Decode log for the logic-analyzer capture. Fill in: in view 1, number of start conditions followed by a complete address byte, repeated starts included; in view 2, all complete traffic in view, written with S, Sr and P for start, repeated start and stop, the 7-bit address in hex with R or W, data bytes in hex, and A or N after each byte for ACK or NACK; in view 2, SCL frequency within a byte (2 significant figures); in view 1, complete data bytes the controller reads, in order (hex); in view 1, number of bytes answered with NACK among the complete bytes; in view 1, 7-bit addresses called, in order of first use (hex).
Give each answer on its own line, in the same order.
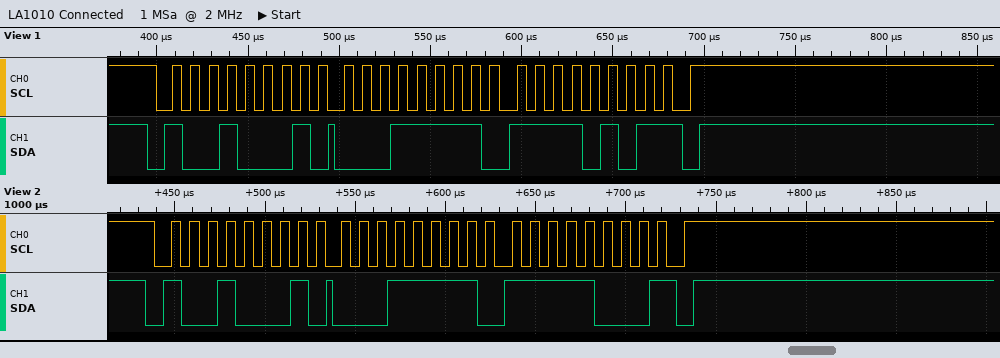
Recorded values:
1
S 48R A 1F A F8 N P
100 kHz
1F F5
1
0x48
